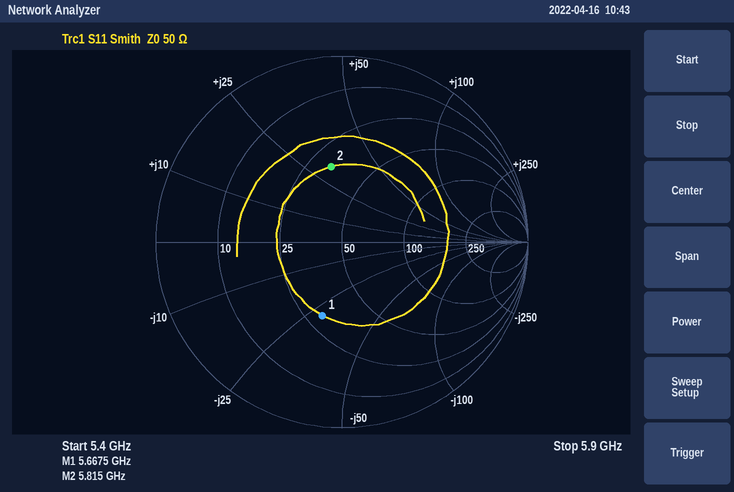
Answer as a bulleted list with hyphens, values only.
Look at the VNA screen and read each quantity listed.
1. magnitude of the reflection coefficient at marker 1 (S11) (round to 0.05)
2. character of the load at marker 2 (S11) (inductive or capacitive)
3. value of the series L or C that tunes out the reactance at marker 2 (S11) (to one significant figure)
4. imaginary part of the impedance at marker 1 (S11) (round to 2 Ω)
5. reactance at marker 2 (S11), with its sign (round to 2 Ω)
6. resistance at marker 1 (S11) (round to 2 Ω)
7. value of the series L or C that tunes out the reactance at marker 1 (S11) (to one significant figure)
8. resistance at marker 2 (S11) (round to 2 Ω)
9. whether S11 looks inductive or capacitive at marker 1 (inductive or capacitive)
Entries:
- 0.40
- inductive
- 900 fF
- -28 Ω
- +32 Ω
- 30 Ω
- 800 pH
- 32 Ω
- capacitive
